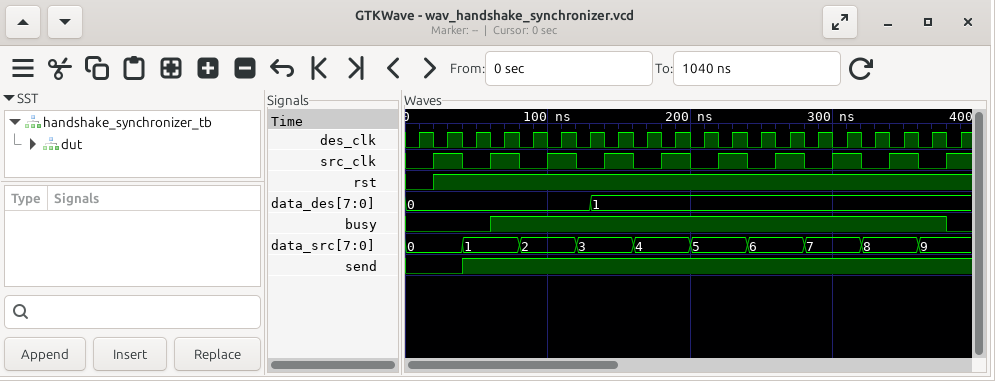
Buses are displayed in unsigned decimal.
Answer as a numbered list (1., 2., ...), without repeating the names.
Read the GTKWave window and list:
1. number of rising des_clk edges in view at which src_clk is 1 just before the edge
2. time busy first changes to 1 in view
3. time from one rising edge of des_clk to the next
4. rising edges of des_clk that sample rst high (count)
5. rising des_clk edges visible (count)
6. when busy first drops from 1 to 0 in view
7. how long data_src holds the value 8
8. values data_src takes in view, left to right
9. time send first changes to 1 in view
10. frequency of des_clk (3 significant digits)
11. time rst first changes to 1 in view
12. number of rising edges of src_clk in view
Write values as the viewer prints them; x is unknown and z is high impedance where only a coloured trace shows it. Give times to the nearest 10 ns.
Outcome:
1. 10
2. 60 ns
3. 20 ns
4. 19
5. 20
6. 380 ns
7. 40 ns
8. 0, 1, 2, 3, 4, 5, 6, 7, 8, 9
9. 40 ns
10. 50.0 MHz
11. 20 ns
12. 10
